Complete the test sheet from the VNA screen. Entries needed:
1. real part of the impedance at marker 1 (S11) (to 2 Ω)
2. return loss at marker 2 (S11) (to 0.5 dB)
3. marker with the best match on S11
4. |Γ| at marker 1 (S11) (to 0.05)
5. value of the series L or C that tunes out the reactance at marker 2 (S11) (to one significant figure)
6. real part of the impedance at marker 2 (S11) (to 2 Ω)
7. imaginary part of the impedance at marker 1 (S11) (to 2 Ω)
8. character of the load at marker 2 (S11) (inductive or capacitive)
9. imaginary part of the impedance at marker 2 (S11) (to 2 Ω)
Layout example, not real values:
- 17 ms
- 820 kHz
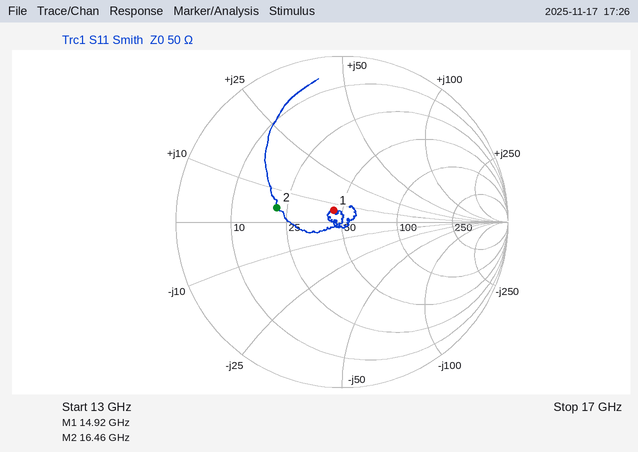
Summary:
- 44 Ω
- 8.0 dB
- marker 1
- 0.10
- 2 pF
- 22 Ω
- +6 Ω
- inductive
- +4 Ω
